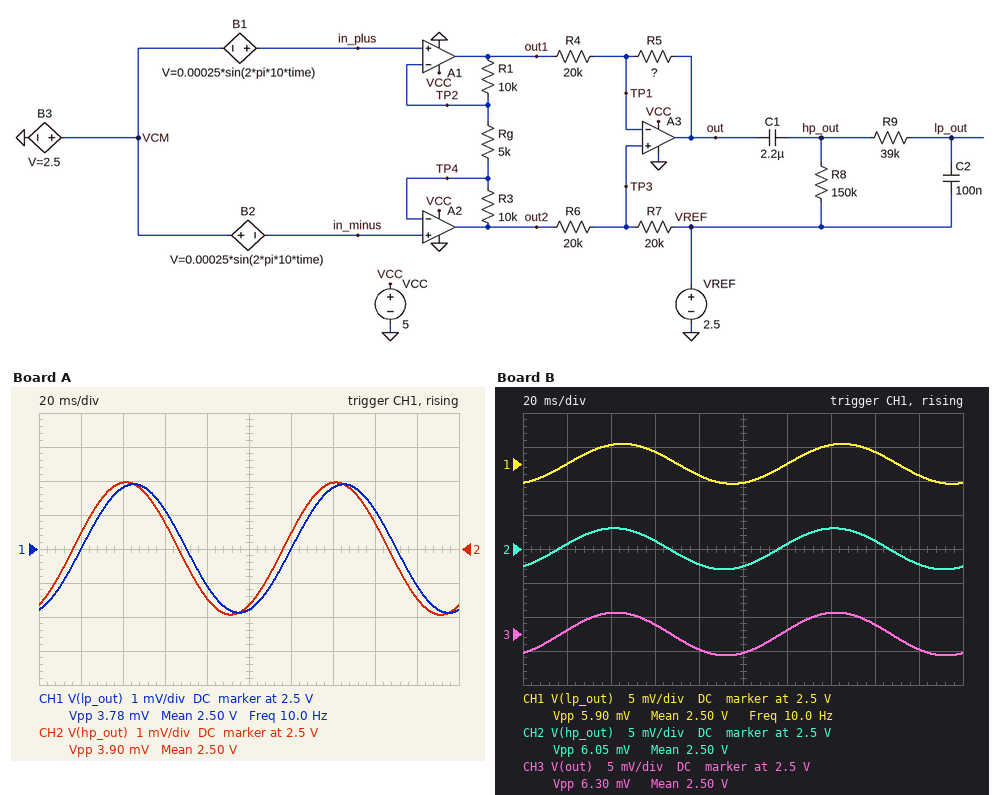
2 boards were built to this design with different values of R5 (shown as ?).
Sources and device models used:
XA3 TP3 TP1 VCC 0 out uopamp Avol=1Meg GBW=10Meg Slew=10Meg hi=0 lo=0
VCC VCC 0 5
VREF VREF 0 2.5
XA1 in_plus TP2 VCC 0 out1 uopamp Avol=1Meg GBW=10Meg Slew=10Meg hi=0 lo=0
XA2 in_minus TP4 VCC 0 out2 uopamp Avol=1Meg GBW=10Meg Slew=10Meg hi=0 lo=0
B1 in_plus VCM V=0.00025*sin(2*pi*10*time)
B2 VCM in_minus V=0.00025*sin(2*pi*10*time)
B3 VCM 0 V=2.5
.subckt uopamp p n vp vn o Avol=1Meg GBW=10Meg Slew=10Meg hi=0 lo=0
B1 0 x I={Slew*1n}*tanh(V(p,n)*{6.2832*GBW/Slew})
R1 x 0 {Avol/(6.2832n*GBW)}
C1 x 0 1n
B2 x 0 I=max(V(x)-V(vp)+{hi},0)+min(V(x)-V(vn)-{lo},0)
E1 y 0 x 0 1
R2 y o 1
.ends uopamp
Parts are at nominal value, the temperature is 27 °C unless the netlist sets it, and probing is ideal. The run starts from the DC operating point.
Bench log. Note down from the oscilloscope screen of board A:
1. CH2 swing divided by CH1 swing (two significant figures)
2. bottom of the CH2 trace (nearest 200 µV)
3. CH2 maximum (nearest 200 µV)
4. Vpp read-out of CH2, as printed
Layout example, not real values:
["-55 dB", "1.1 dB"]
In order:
["1.0", "2.4980 V", "2.5020 V", "3.90 mV"]
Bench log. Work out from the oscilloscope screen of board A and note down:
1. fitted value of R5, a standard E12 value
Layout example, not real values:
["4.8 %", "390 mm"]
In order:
["15 kΩ"]
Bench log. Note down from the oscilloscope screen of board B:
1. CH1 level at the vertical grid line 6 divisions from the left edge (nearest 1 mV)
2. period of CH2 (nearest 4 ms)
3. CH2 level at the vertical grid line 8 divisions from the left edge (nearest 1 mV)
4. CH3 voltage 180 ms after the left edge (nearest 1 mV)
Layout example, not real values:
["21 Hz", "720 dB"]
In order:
["2.500 V", "100 ms", "2.501 V", "2.498 V"]
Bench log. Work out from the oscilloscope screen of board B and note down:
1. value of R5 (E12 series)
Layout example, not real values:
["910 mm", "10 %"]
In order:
["27 kΩ"]
